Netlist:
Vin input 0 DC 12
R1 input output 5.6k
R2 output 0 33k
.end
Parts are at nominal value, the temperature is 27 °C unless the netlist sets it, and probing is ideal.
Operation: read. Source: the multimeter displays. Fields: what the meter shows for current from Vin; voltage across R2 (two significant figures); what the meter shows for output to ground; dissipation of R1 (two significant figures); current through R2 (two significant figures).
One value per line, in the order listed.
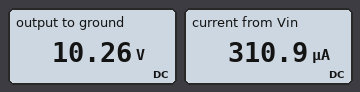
310.9 µA
10 V
10.26 V
540 µW
310 µA
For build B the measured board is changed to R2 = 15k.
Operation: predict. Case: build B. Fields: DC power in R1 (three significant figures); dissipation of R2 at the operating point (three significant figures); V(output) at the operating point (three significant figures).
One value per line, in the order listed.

1.90 mW
5.09 mW
8.74 V
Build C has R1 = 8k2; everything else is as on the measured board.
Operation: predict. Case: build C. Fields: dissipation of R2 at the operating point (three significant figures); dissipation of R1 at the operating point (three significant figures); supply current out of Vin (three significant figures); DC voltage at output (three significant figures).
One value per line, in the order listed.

2.80 mW
696 µW
291 µA
9.61 V
